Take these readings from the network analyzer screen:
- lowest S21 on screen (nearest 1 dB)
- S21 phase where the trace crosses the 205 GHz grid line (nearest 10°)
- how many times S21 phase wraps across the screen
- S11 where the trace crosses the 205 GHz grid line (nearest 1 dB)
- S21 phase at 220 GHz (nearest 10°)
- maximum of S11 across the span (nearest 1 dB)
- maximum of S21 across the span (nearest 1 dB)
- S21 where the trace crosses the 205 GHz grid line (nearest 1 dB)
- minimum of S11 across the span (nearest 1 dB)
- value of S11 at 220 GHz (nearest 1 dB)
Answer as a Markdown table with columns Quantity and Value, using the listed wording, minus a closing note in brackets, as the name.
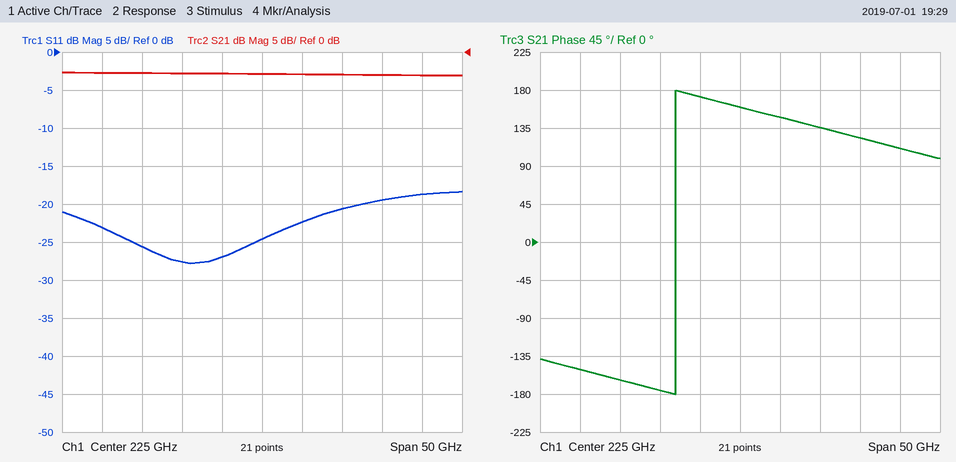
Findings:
| Quantity | Value |
|---|---|
| lowest S21 on screen | -3 dB |
| S21 phase where the trace crosses the 205 GHz grid line | -150° |
| how many times S21 phase wraps across the screen | 1 |
| S11 where the trace crosses the 205 GHz grid line | -23 dB |
| S21 phase at 220 GHz | 170° |
| maximum of S11 across the span | -18 dB |
| maximum of S21 across the span | -3 dB |
| S21 where the trace crosses the 205 GHz grid line | -3 dB |
| minimum of S11 across the span | -28 dB |
| value of S11 at 220 GHz | -27 dB |
